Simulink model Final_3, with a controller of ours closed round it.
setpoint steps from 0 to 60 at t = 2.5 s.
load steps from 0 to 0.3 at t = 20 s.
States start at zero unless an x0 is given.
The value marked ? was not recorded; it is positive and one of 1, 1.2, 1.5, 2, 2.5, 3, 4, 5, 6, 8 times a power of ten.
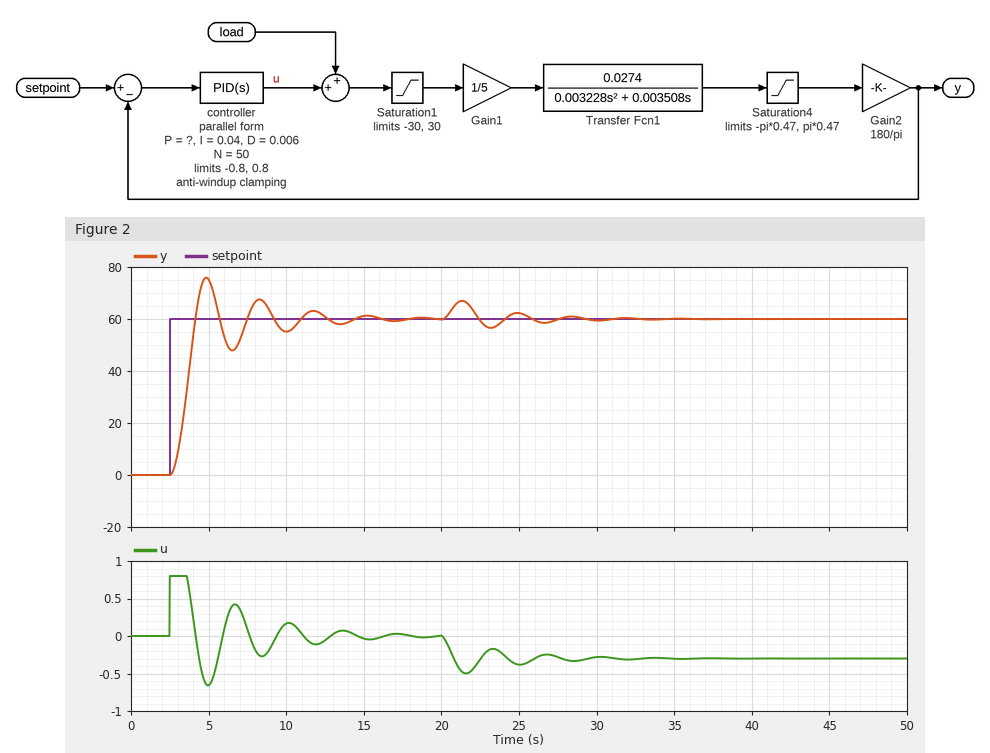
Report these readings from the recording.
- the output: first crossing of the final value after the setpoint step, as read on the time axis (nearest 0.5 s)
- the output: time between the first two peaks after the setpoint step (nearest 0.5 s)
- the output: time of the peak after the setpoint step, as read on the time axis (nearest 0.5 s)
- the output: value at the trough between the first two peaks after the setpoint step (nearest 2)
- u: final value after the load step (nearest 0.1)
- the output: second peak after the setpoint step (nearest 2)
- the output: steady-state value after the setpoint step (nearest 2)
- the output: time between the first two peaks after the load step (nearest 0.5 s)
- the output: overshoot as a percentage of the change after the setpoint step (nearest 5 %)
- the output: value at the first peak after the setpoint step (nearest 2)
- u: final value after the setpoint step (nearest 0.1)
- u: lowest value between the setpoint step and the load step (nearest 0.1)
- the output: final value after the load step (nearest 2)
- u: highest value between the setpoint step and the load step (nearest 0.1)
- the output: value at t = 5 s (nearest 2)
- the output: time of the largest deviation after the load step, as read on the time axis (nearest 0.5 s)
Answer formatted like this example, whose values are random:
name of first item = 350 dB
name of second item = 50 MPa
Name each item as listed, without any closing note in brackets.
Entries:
the output: first crossing of the final value after the setpoint step, as read on the time axis = 4.0 s
the output: time between the first two peaks after the setpoint step = 3.5 s
the output: time of the peak after the setpoint step, as read on the time axis = 5.0 s
the output: value at the trough between the first two peaks after the setpoint step = 48
u: final value after the load step = -0.3
the output: second peak after the setpoint step = 68
the output: steady-state value after the setpoint step = 60
the output: time between the first two peaks after the load step = 3.5 s
the output: overshoot as a percentage of the change after the setpoint step = 25 %
the output: value at the first peak after the setpoint step = 76
u: final value after the setpoint step = 0.0
u: lowest value between the setpoint step and the load step = -0.7
the output: final value after the load step = 60
u: highest value between the setpoint step and the load step = 0.8
the output: value at t = 5 s = 76
the output: time of the largest deviation after the load step, as read on the time axis = 21.5 s
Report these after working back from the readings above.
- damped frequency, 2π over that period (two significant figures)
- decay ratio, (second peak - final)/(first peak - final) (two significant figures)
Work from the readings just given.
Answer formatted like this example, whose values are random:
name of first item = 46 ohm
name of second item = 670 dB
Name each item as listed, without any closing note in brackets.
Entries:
damped frequency, 2π over that period = 1.8 rad/s
decay ratio, (second peak - final)/(first peak - final) = 0.50
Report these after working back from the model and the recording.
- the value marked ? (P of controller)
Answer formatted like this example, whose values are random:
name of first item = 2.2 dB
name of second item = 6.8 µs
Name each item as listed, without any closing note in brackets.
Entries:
the value marked ? = 0.04
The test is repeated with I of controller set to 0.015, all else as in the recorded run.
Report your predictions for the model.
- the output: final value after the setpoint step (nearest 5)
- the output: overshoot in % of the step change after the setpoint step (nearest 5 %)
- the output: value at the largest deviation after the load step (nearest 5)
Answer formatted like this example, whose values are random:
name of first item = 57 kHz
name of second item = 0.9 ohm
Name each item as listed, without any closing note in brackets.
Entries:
the output: final value after the setpoint step = 60
the output: overshoot in % of the step change after the setpoint step = 20 %
the output: value at the largest deviation after the load step = 70
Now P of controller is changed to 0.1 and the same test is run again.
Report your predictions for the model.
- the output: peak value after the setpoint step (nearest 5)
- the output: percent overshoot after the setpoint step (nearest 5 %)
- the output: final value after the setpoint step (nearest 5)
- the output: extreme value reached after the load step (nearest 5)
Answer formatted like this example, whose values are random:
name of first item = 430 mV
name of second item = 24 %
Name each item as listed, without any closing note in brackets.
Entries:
the output: peak value after the setpoint step = 70
the output: percent overshoot after the setpoint step = 20 %
the output: final value after the setpoint step = 60
the output: extreme value reached after the load step = 65
